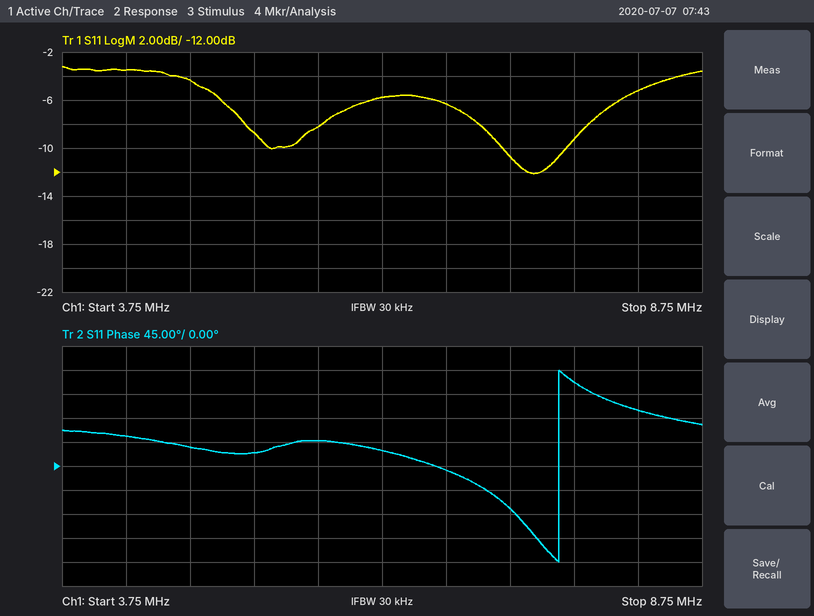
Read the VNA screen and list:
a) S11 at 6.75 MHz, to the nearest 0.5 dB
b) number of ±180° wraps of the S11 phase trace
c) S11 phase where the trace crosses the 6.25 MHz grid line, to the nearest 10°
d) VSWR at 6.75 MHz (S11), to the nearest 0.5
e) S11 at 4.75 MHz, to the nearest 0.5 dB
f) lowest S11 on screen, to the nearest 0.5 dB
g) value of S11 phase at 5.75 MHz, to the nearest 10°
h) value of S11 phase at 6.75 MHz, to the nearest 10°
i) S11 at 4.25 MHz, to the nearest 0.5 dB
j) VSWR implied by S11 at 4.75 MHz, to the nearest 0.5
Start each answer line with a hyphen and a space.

- -6.5 dB
- 1
- 30°
- 3.0
- -4.5 dB
- -12.0 dB
- 50°
- -10°
- -3.5 dB
- 4.0
